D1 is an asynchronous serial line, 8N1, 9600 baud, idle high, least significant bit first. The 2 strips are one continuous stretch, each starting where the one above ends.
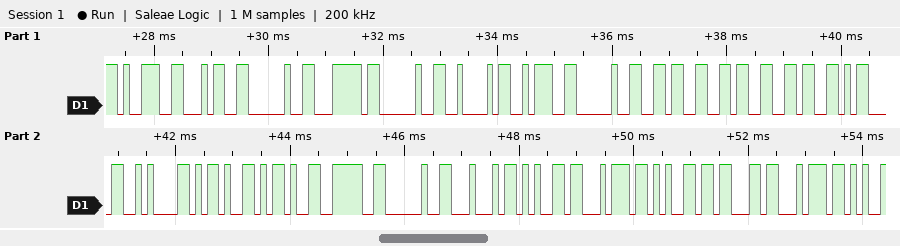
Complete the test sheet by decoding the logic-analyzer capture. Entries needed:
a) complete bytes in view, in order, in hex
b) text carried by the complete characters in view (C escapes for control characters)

0x39 0x34 0x20 0x7C 0x20 0x42 0x3A 0x20 0x36 0x36 0x36 0x0D 0x0A 0x2D 0x2D 0x3E 0x20 0x44 0x65 0x74 0x65 0x63 0x74
"94 | B: 666\r\n--> Detect"
